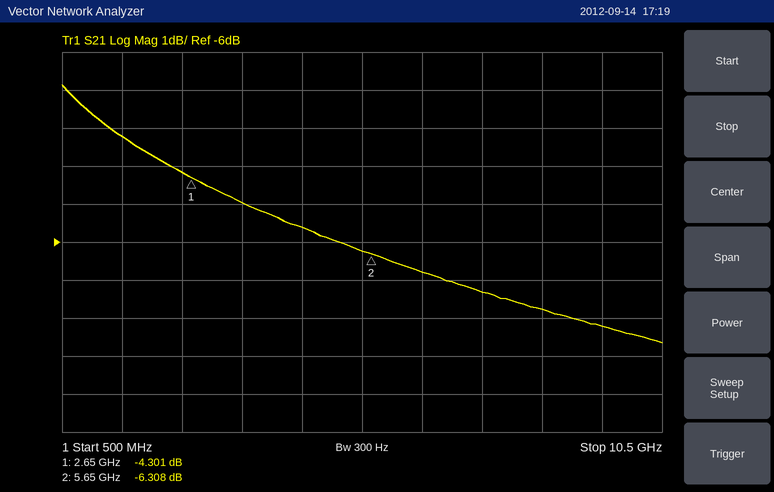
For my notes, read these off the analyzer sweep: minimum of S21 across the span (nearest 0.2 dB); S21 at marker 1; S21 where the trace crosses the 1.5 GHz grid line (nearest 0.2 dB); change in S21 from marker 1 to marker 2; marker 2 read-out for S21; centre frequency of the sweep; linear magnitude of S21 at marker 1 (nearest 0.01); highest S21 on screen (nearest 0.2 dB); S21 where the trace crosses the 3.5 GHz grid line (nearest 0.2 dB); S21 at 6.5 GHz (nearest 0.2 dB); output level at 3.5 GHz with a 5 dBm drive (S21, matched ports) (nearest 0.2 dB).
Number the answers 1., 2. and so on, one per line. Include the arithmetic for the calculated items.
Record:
1. -8.6 dB
2. -4.301 dB
3. -3.2 dB
4. -6.308 − (-4.301) = -2.007 dB
5. -6.308 dB
6. 5.5 GHz
7. 10^(-4.301/20) ≈ 0.61
8. -1.8 dB
9. -5.0 dB
10. -6.8 dB
11. 5 dBm + (-5.0 dB) = 0.0 dBm
